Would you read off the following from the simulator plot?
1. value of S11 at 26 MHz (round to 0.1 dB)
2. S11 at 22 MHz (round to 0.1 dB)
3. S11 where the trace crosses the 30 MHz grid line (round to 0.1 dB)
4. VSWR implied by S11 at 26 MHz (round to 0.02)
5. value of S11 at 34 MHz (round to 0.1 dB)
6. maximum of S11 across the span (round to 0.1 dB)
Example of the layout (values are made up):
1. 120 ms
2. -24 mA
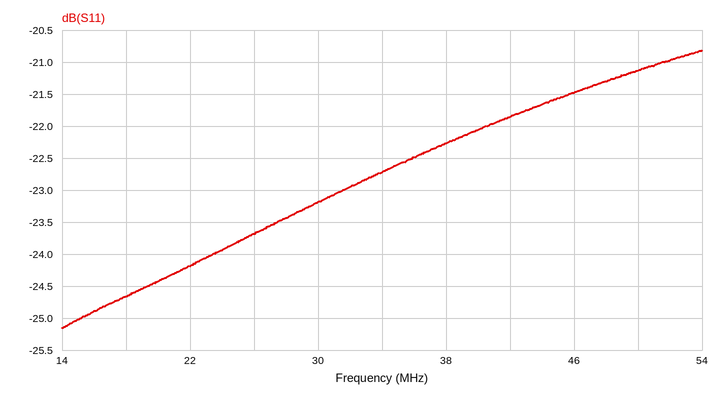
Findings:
1. -23.7 dB
2. -24.2 dB
3. -23.2 dB
4. 1.14
5. -22.7 dB
6. -20.8 dB
